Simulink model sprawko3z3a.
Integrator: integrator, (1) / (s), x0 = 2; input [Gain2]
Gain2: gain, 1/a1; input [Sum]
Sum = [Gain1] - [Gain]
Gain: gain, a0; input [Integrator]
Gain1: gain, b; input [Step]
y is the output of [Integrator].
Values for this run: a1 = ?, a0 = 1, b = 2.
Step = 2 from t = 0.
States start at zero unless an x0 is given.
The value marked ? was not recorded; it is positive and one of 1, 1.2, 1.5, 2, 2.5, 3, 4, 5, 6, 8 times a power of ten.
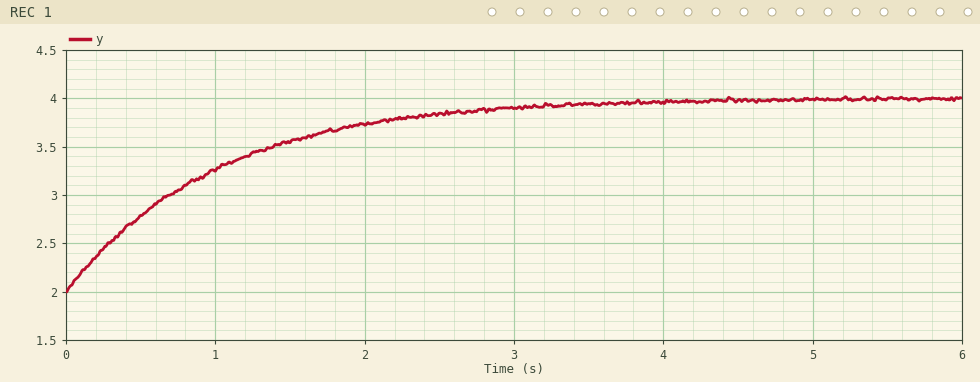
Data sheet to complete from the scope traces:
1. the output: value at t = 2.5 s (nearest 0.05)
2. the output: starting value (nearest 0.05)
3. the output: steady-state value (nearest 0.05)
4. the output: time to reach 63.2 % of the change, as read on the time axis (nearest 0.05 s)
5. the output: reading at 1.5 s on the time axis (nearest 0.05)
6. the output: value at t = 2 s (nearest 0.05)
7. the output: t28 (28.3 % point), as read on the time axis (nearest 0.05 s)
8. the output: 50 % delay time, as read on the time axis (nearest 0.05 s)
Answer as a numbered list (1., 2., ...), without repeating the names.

1. 3.85
2. 2.00
3. 4.00
4. 1.00 s
5. 3.55
6. 3.75
7. 0.35 s
8. 0.70 s
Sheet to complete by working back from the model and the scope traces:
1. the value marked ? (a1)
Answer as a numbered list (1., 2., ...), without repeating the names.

1. 1
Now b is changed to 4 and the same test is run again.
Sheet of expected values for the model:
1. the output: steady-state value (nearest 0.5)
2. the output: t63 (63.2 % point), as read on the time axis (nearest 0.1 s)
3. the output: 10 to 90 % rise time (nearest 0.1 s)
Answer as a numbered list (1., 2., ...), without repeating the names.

1. 8.0
2. 1.0 s
3. 2.2 s
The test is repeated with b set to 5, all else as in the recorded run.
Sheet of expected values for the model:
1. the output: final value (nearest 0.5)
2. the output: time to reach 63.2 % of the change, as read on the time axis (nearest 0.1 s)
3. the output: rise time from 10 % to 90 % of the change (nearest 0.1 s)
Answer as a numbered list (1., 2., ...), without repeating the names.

1. 10.0
2. 1.0 s
3. 2.2 s
